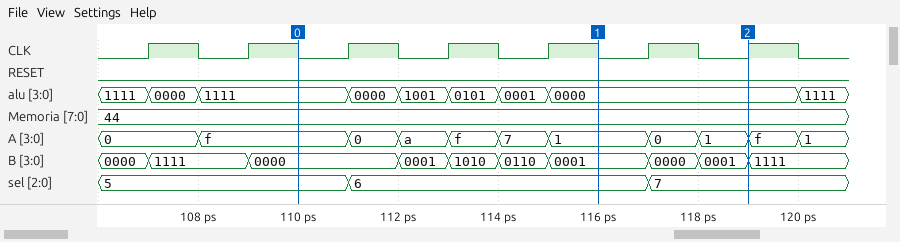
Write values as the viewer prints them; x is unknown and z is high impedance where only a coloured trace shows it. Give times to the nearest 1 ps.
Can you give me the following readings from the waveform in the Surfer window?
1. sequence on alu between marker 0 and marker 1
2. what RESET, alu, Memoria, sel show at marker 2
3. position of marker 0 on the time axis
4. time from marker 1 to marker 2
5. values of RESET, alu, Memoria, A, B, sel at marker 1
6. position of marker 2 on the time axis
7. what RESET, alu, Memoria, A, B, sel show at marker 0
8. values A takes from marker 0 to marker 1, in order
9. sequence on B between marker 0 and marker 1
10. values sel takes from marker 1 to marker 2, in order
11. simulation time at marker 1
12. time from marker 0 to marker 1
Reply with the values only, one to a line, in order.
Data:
1111, 0000, 1001, 0101, 0001, 0000
RESET=0, alu=0000, Memoria=44, sel=7
110 ps
3 ps
RESET=0, alu=0000, Memoria=44, A=1, B=0001, sel=6
119 ps
RESET=0, alu=1111, Memoria=44, A=f, B=0000, sel=5
f, 0, a, f, 7, 1
0000, 0001, 1010, 0110, 0001
6, 7
116 ps
6 ps
